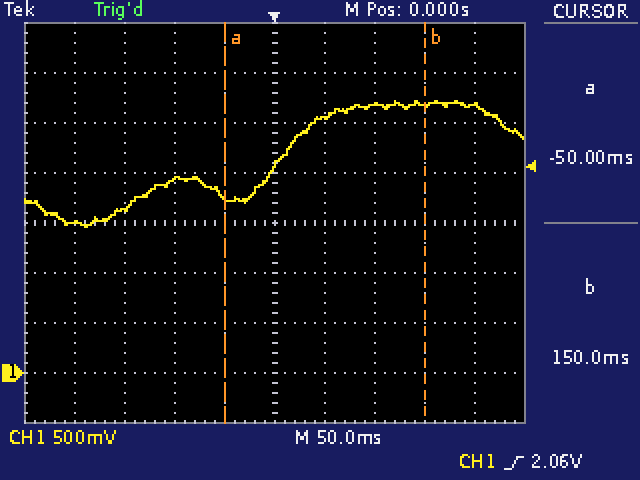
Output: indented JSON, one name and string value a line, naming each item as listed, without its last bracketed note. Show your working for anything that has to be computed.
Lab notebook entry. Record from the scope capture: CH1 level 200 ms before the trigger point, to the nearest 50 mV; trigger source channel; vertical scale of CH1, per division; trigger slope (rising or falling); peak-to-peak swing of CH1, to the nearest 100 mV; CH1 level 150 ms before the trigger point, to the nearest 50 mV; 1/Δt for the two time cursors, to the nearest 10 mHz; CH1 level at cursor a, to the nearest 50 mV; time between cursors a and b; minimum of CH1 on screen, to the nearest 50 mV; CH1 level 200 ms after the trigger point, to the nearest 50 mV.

{
  "CH1 level 200 ms before the trigger point, to the nearest 50 mV": "1.50 V",
  "trigger source channel": "CH1",
  "vertical scale of CH1, per division": "500 mV",
  "trigger slope": "rising",
  "peak-to-peak swing of CH1, to the nearest 100 mV": "1.30 V",
  "CH1 level 150 ms before the trigger point, to the nearest 50 mV": "1.65 V",
  "1/Δt for the two time cursors, to the nearest 10 mHz": "1 / 200 ms ≈ 5.00 Hz",
  "CH1 level at cursor a, to the nearest 50 mV": "1.75 V",
  "time between cursors a and b": "150 ms − (-50 ms) = 200 ms",
  "minimum of CH1 on screen, to the nearest 50 mV": "1.45 V",
  "CH1 level 200 ms after the trigger point, to the nearest 50 mV": "2.70 V"
}
